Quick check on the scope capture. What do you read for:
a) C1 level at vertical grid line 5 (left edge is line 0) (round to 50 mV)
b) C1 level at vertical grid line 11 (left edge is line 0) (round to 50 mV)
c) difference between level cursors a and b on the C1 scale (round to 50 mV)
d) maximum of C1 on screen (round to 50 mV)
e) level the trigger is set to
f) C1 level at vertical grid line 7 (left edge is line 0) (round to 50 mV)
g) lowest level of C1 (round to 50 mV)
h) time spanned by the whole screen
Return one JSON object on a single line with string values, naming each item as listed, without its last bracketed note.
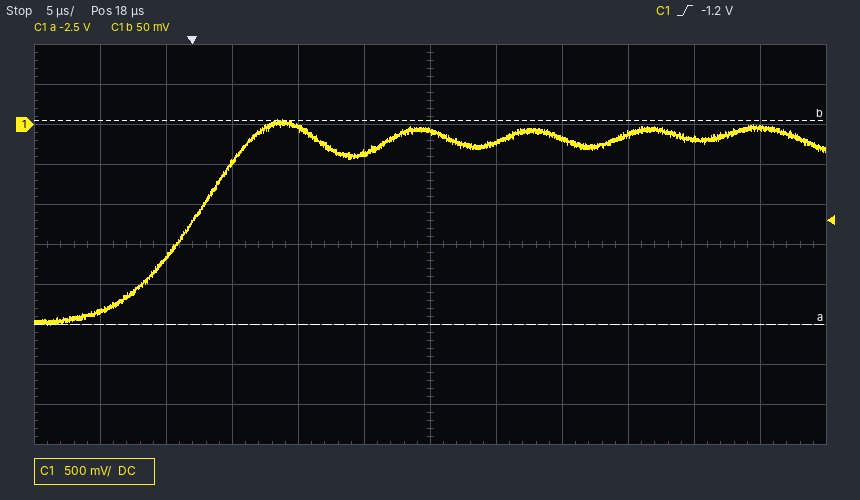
{"C1 level at vertical grid line 5 (left edge is line 0)": "-350 mV", "C1 level at vertical grid line 11 (left edge is line 0)": "-50 mV", "difference between level cursors a and b on the C1 scale": "2.55 V", "maximum of C1 on screen": "50 mV", "level the trigger is set to": "-1.2 V", "C1 level at vertical grid line 7 (left edge is line 0)": "-250 mV", "lowest level of C1": "-2.50 V", "time spanned by the whole screen": "60 µs"}
